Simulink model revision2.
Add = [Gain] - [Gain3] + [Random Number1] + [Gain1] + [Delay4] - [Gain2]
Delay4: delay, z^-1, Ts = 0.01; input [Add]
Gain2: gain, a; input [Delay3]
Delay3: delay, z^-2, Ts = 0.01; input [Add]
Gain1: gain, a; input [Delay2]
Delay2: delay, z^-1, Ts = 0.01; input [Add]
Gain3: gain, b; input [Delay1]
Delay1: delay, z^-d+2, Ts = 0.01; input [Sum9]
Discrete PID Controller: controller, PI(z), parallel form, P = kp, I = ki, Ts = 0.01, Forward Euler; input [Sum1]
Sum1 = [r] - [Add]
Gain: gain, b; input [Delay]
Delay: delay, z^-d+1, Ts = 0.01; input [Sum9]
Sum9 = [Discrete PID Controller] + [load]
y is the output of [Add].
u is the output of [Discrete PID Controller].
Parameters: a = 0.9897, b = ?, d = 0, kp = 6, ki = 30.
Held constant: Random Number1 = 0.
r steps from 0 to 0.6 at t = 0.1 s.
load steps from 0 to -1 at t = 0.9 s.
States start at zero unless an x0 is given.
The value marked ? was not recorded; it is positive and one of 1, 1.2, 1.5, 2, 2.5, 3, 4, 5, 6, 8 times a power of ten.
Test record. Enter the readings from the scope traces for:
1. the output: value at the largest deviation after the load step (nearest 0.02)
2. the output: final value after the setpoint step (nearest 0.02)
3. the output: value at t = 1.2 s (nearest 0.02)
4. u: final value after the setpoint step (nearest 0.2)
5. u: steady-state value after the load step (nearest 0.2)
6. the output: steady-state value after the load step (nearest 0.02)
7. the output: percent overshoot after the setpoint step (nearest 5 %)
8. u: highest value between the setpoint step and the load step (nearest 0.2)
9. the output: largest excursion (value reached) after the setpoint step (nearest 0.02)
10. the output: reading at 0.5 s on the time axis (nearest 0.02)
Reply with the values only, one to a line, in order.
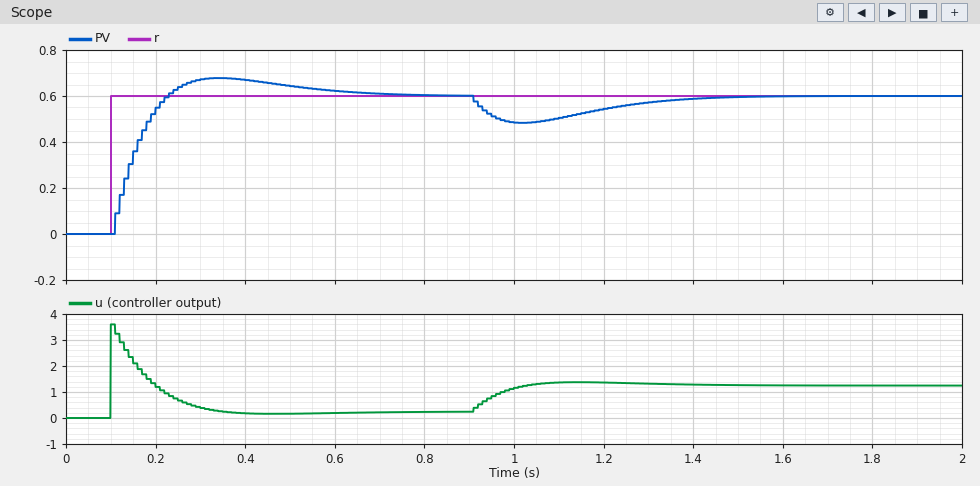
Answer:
0.48
0.60
0.54
0.2
1.2
0.60
15 %
3.6
0.68
0.64
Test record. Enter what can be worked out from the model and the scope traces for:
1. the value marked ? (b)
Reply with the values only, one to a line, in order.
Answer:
0.025
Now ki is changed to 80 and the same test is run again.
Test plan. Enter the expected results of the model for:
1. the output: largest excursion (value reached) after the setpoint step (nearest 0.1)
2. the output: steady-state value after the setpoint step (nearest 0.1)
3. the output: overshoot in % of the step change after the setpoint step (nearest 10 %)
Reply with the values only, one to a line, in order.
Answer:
0.8
0.6
30 %
